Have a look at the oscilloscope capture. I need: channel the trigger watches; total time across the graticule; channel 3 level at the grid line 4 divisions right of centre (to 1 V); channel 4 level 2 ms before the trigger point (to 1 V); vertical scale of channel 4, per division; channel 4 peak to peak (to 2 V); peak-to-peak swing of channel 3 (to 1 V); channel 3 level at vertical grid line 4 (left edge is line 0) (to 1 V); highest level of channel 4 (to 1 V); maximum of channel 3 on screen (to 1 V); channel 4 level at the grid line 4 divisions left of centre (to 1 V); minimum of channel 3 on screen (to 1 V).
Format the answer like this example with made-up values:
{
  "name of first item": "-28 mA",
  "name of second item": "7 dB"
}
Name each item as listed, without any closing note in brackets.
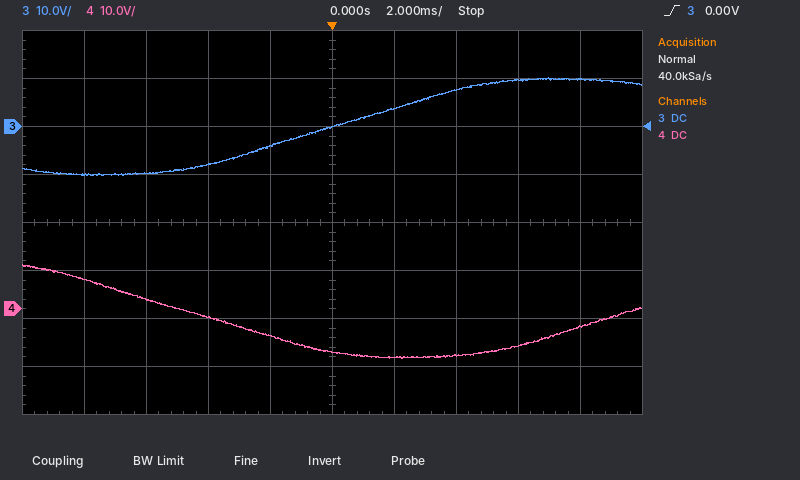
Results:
{
  "channel the trigger watches": "channel 3",
  "total time across the graticule": "20 ms",
  "channel 3 level at the grid line 4 divisions right of centre": "10 V",
  "channel 4 level 2 ms before the trigger point": "-6 V",
  "vertical scale of channel 4, per division": "10 V",
  "channel 4 peak to peak": "20 V",
  "peak-to-peak swing of channel 3": "20 V",
  "channel 3 level at vertical grid line 4 (left edge is line 0)": "-4 V",
  "highest level of channel 4": "9 V",
  "maximum of channel 3 on screen": "10 V",
  "channel 4 level at the grid line 4 divisions left of centre": "6 V",
  "minimum of channel 3 on screen": "-10 V"
}
